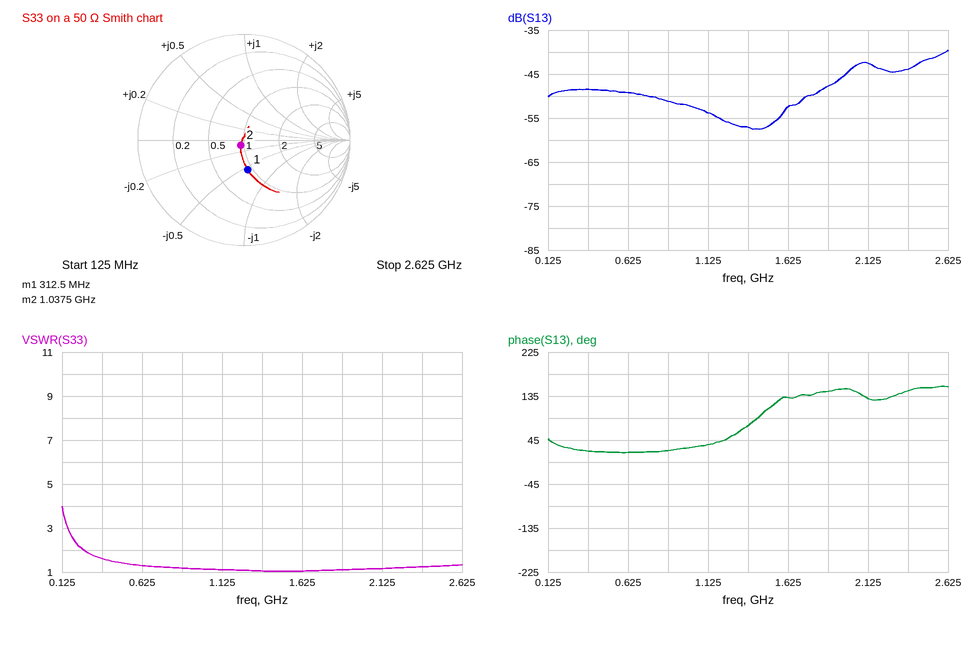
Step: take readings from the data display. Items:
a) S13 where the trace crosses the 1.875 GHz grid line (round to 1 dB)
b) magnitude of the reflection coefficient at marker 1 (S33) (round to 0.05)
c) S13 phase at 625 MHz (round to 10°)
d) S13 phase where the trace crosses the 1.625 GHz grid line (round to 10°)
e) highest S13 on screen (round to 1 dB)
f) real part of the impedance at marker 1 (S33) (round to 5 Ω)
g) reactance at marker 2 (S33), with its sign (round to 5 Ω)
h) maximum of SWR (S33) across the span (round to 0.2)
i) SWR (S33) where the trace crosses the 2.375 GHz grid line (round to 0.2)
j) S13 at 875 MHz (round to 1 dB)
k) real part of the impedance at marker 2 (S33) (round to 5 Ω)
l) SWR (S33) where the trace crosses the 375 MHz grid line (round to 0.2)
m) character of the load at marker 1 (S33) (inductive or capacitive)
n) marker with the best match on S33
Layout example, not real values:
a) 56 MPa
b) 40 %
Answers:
a) -48 dB
b) 0.30
c) 20°
d) 130°
e) -40 dB
f) 45 Ω
g) -5 Ω
h) 4.0
i) 1.2
j) -51 dB
k) 45 Ω
l) 1.6
m) capacitive
n) marker 2
